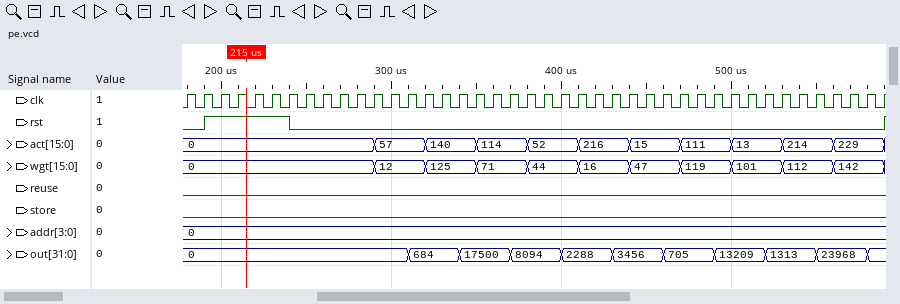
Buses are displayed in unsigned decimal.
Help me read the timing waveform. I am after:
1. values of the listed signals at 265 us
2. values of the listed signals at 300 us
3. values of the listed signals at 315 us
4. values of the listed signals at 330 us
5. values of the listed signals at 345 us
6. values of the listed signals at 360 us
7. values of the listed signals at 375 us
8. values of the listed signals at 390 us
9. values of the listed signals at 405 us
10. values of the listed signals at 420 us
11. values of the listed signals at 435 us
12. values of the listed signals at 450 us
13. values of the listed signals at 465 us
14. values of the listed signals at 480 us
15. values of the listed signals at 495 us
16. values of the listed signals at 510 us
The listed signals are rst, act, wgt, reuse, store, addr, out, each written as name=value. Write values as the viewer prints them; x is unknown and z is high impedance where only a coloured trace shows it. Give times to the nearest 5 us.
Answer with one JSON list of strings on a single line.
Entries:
["rst=0, act=0, wgt=0, reuse=0, store=0, addr=0, out=0", "rst=0, act=57, wgt=12, reuse=0, store=0, addr=0, out=0", "rst=0, act=57, wgt=12, reuse=0, store=0, addr=0, out=684", "rst=0, act=140, wgt=125, reuse=0, store=0, addr=0, out=684", "rst=0, act=140, wgt=125, reuse=0, store=0, addr=0, out=17500", "rst=0, act=114, wgt=71, reuse=0, store=0, addr=0, out=17500", "rst=0, act=114, wgt=71, reuse=0, store=0, addr=0, out=8094", "rst=0, act=52, wgt=44, reuse=0, store=0, addr=0, out=8094", "rst=0, act=52, wgt=44, reuse=0, store=0, addr=0, out=2288", "rst=0, act=216, wgt=16, reuse=0, store=0, addr=0, out=2288", "rst=0, act=216, wgt=16, reuse=0, store=0, addr=0, out=3456", "rst=0, act=15, wgt=47, reuse=0, store=0, addr=0, out=3456", "rst=0, act=15, wgt=47, reuse=0, store=0, addr=0, out=705", "rst=0, act=111, wgt=119, reuse=0, store=0, addr=0, out=705", "rst=0, act=111, wgt=119, reuse=0, store=0, addr=0, out=13209", "rst=0, act=13, wgt=101, reuse=0, store=0, addr=0, out=13209"]
